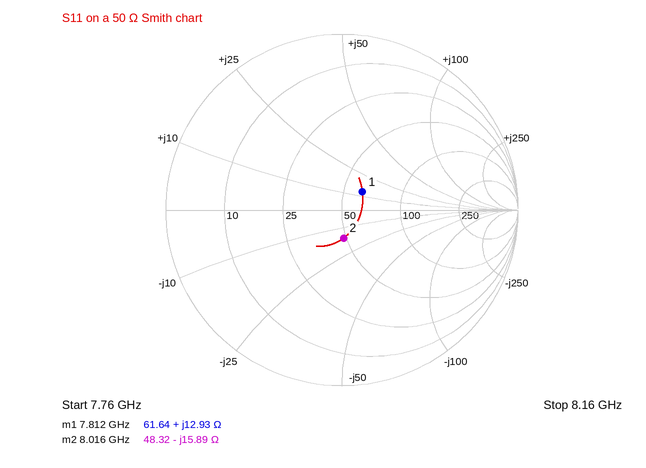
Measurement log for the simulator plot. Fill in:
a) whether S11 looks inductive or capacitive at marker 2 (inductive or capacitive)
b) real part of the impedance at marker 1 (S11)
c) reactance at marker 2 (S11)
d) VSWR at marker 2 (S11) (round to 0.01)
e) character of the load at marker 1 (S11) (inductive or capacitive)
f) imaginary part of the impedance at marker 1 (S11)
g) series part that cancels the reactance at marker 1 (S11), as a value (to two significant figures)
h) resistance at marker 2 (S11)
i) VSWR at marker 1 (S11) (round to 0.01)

capacitive
61.64 Ω
-15.89 Ω
1.38
inductive
+12.93 Ω
1.6 pF
48.32 Ω
1.37
